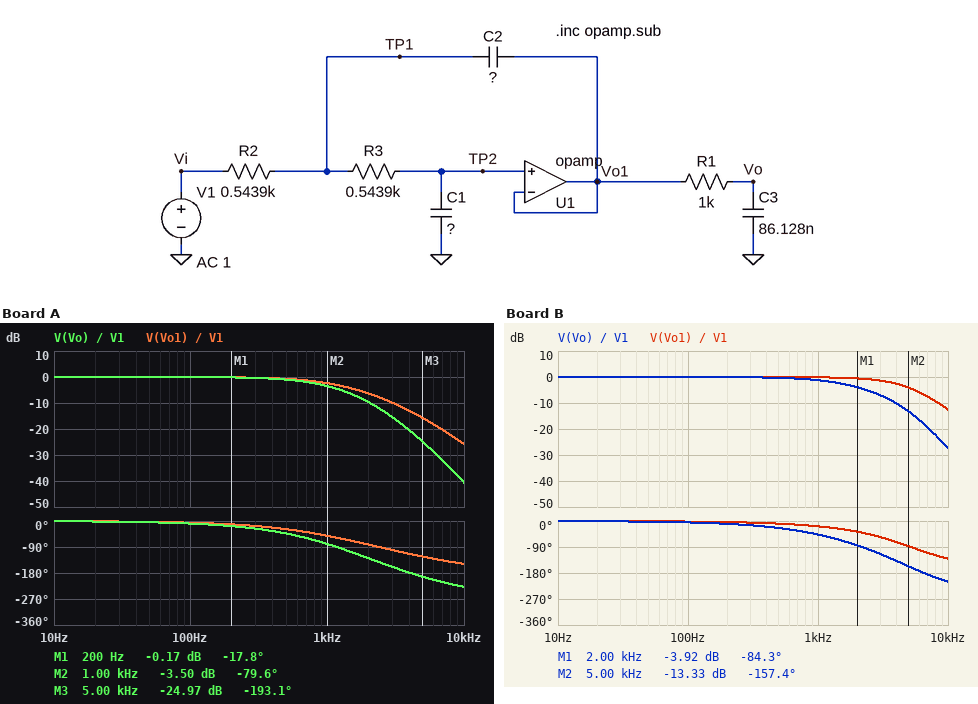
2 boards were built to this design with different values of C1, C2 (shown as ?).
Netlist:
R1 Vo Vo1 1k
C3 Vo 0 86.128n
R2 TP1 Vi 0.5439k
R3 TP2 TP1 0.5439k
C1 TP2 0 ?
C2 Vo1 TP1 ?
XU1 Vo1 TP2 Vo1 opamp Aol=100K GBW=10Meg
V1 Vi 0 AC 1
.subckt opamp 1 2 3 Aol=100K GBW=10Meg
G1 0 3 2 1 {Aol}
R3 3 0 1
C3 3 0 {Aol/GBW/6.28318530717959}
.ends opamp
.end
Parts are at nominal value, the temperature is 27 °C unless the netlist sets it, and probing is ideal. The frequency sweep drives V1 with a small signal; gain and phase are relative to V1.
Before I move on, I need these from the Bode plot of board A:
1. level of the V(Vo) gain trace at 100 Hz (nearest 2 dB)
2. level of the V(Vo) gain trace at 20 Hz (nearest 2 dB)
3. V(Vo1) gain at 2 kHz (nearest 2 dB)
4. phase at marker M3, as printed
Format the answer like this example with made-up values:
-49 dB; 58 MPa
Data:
0 dB; 0 dB; -6 dB; -193.1 deg
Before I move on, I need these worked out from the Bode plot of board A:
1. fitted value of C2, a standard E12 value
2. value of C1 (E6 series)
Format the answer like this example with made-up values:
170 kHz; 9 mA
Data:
100 nF; 150 nF
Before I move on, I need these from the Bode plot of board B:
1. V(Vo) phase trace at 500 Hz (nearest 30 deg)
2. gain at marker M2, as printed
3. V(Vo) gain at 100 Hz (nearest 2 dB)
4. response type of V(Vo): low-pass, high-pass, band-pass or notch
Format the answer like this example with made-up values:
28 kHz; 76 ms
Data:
-30 deg; -13.33 dB; 0 dB; low-pass
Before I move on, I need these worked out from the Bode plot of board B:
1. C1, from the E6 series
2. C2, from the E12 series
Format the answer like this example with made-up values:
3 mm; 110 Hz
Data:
47 nF; 68 nF
